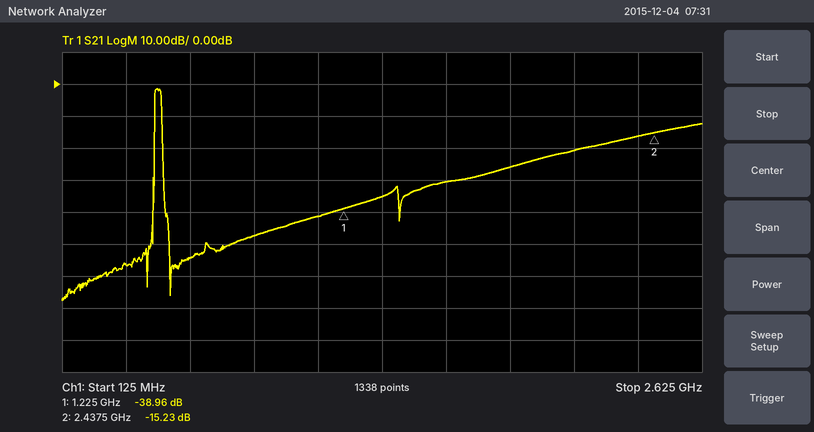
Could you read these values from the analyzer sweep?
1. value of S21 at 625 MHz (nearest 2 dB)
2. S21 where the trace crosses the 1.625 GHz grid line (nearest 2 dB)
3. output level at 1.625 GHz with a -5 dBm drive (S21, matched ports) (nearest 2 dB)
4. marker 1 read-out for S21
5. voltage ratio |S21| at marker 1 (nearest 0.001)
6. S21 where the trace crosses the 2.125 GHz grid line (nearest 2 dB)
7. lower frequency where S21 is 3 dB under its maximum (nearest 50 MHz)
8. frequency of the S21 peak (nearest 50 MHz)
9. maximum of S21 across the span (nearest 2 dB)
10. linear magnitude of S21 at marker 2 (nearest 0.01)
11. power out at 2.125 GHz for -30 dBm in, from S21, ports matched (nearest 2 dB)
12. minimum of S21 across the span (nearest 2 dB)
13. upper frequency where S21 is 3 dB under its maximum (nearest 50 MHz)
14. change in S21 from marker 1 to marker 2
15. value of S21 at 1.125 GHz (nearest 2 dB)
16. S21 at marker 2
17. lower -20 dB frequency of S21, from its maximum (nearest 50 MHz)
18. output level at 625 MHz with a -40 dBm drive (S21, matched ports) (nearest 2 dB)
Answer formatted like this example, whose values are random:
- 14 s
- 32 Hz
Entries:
- -54 dB
- -30 dB
- -36 dBm
- -38.96 dB
- 0.011
- -20 dB
- 500 MHz
- 500 MHz
- -2 dB
- 0.17
- -50 dBm
- -68 dB
- 500 MHz
- 23.73 dB
- -42 dB
- -15.23 dB
- 500 MHz
- -94 dBm
